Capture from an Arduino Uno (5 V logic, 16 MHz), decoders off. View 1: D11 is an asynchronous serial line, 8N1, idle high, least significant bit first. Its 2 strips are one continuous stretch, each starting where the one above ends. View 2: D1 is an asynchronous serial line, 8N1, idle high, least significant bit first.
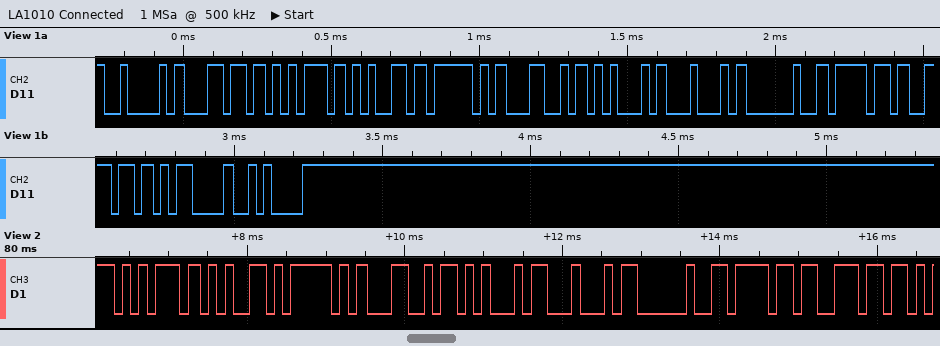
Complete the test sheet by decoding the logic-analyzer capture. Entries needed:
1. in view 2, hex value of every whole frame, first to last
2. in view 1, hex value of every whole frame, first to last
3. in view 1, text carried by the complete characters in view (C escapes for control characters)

0x75 0x65 0x5F 0x4C 0x45 0x44 0x20 0x6F 0x6E
42 6C 75 65 5F 4C 45 44 20 6F 6E 0D 0A
"Blue_LED on\r\n"
